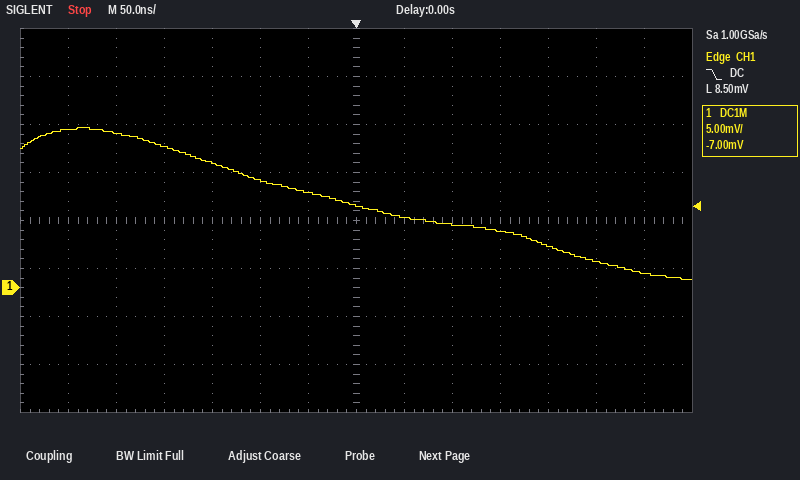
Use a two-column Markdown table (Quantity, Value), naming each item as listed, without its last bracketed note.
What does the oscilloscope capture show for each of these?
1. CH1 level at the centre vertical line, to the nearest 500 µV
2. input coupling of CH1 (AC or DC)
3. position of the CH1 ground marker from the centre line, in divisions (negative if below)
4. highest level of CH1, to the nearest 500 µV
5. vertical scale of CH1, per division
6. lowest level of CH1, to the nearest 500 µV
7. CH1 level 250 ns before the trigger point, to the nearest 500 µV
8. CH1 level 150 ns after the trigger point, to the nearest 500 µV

| Quantity | Value |
|---|---|
| CH1 level at the centre vertical line, to the nearest 500 µV | 8.5 mV |
| input coupling of CH1 | DC |
| position of the CH1 ground marker from the centre line, in divisions | -1.4 div |
| highest level of CH1, to the nearest 500 µV | 16.5 mV |
| vertical scale of CH1, per division | 5 mV |
| lowest level of CH1, to the nearest 500 µV | 1.0 mV |
| CH1 level 250 ns before the trigger point, to the nearest 500 µV | 16.0 mV |
| CH1 level 150 ns after the trigger point, to the nearest 500 µV | 6.0 mV |
